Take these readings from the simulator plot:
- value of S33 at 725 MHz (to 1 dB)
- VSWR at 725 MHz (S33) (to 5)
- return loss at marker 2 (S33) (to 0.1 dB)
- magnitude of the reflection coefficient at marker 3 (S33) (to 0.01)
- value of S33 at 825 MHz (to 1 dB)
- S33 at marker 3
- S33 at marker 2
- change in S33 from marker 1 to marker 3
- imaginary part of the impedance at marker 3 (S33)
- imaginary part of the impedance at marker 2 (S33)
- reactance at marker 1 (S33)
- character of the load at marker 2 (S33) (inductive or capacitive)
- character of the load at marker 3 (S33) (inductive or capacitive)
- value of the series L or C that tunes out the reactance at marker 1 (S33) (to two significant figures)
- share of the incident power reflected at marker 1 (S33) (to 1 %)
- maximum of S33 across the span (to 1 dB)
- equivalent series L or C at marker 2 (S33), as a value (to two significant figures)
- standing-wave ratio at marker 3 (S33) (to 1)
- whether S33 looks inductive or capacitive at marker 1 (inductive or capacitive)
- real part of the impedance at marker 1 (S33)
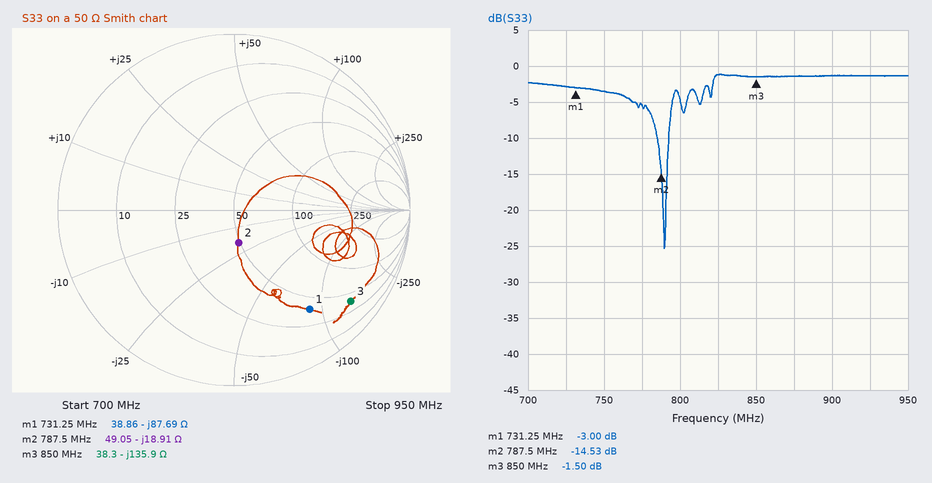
-3 dB
5
14.5 dB
0.84
-1 dB
-1.50 dB
-14.53 dB
1.50 dB
-135.9 Ω
-18.91 Ω
-87.69 Ω
capacitive
capacitive
19 nH
50 %
-1 dB
11 pF
12
capacitive
38.86 Ω
